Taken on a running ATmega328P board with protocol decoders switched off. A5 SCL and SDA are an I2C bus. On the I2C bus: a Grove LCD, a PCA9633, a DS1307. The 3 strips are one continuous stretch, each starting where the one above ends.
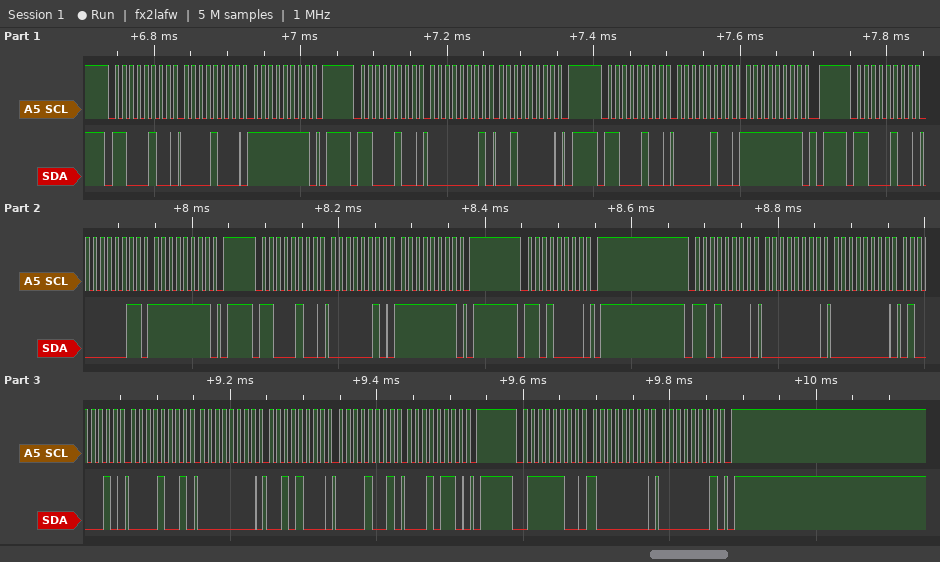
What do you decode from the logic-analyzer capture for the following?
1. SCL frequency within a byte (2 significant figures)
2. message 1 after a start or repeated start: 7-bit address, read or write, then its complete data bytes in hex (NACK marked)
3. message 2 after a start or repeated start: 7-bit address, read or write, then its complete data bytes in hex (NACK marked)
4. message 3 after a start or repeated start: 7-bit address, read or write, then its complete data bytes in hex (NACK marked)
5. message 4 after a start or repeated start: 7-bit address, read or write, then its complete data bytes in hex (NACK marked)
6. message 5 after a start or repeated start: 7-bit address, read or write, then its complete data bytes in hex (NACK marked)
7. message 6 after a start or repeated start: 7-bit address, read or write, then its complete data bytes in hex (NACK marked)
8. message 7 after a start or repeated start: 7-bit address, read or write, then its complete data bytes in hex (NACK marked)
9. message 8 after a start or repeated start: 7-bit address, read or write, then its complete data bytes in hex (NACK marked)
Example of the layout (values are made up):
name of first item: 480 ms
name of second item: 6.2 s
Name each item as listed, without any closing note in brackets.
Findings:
SCL frequency within a byte: 100 kHz
message 1 after a start or repeated start: 7-bit address, read or write, then its complete data bytes in hex: 0x62 write: 08 FF
message 2 after a start or repeated start: 7-bit address, read or write, then its complete data bytes in hex: 0x62 write: 01 20
message 3 after a start or repeated start: 7-bit address, read or write, then its complete data bytes in hex: 0x62 write: 04 FF
message 4 after a start or repeated start: 7-bit address, read or write, then its complete data bytes in hex: 0x62 write: 03 FF
message 5 after a start or repeated start: 7-bit address, read or write, then its complete data bytes in hex: 0x62 write: 02 FF
message 6 after a start or repeated start: 7-bit address, read or write, then its complete data bytes in hex: 0x68 write
message 7 after a start or repeated start: 7-bit address, read or write, then its complete data bytes in hex: 0x68 write: 00 00 42 09 00 28 09 16
message 8 after a start or repeated start: 7-bit address, read or write, then its complete data bytes in hex: 0x3E write: 80 01
